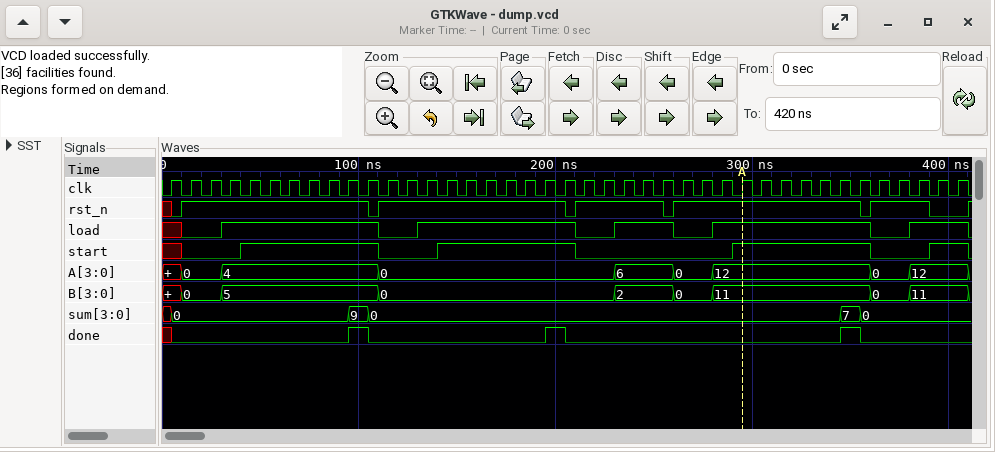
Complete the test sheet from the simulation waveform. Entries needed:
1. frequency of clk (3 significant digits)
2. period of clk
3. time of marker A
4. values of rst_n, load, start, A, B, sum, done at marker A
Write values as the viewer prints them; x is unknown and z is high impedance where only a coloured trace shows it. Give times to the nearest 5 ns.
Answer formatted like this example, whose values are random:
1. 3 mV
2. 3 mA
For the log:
1. 100 MHz
2. 10 ns
3. 295 ns
4. rst_n=1, load=1, start=1, A=12, B=11, sum=0, done=0
